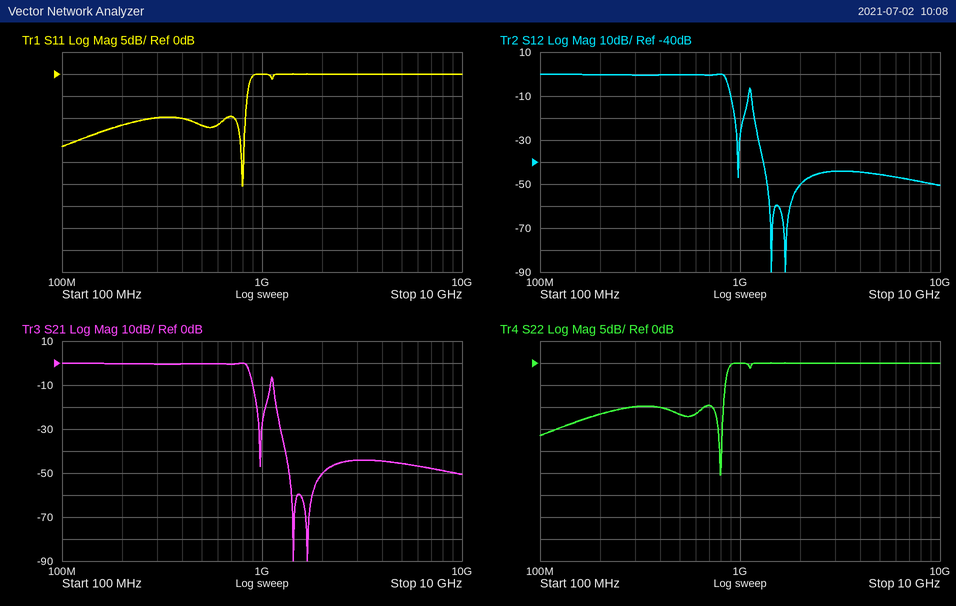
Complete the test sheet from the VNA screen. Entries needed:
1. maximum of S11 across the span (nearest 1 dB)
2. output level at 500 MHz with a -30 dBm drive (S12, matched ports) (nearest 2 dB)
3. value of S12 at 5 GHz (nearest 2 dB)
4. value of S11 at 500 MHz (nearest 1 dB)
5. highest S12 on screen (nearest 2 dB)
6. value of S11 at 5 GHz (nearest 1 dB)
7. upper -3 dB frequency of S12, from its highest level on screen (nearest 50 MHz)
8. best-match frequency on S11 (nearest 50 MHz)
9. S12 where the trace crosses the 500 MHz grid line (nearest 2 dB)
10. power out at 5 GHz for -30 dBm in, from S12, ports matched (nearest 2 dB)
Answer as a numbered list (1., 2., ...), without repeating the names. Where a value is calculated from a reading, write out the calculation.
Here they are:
1. 0 dB
2. -30 dBm + (0 dB) = -30 dBm
3. -46 dB
4. -12 dB
5. 0 dB
6. 0 dB
7. 850 MHz
8. 800 MHz
9. 0 dB
10. -30 dBm + (-46 dB) = -76 dBm
